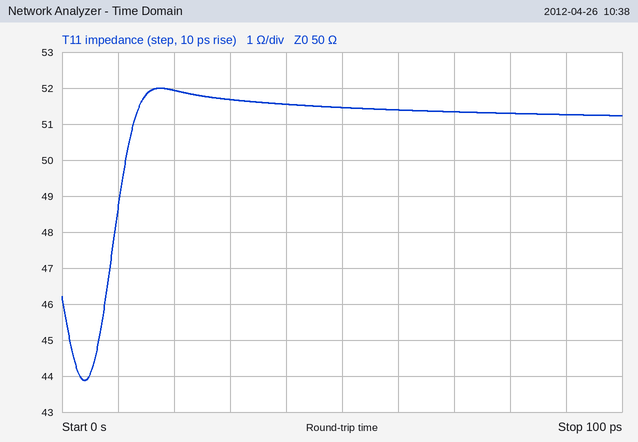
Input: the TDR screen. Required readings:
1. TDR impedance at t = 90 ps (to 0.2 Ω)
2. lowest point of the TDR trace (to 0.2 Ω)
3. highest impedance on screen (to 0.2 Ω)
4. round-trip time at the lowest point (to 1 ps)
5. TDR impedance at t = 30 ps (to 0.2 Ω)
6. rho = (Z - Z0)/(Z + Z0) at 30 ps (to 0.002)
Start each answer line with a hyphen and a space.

- 51.2 Ω
- 43.8 Ω
- 52.0 Ω
- 4 ps
- 51.6 Ω
- +0.016
